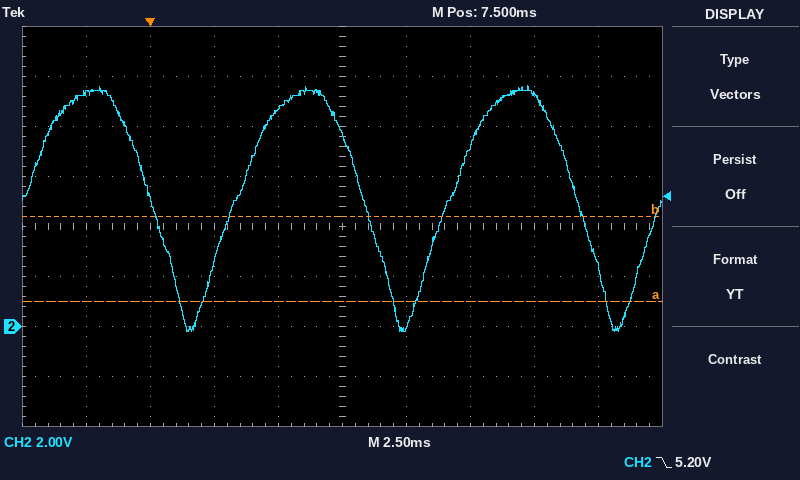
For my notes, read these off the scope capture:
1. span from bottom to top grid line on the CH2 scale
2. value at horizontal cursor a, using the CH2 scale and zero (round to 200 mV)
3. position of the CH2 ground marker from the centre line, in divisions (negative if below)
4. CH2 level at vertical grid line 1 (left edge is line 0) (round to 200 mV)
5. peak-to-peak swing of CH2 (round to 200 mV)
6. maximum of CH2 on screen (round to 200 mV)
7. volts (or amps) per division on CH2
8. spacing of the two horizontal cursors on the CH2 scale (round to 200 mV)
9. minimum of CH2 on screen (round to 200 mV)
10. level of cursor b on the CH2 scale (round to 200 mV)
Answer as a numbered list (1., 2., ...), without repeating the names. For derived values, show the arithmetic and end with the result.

1. 16 V
2. 1.0 V
3. -2.0 div
4. 9.4 V
5. 9.6 V − (-200 mV) = 9.8 V
6. 9.6 V
7. 2 V
8. 3.4 V
9. -200 mV
10. 4.4 V
